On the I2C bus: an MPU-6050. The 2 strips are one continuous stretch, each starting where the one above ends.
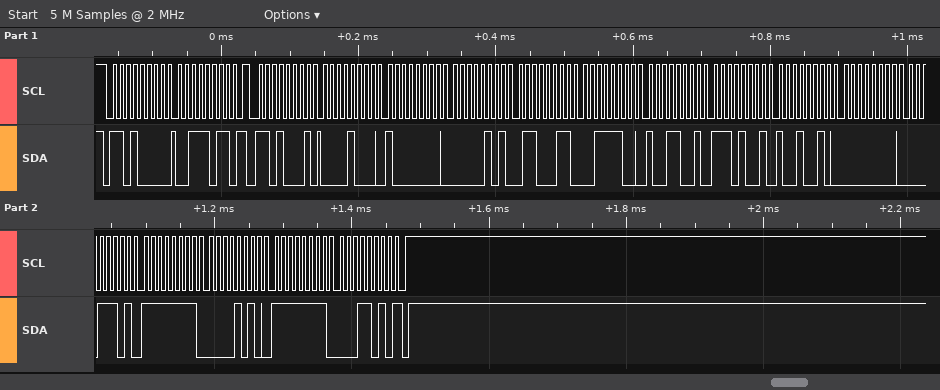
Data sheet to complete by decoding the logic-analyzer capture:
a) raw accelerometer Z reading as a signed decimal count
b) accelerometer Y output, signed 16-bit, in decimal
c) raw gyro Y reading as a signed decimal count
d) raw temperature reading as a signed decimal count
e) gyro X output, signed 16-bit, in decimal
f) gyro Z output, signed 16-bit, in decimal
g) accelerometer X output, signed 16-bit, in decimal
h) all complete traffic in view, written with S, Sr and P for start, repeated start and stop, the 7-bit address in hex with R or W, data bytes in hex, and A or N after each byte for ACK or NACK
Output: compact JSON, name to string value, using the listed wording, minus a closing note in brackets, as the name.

{"raw accelerometer Z reading as a signed decimal count": "15513", "accelerometer Y output, signed 16-bit, in decimal": "1379", "raw gyro Y reading as a signed decimal count": "-246", "raw temperature reading as a signed decimal count": "-5742", "gyro X output, signed 16-bit, in decimal": "29", "gyro Z output, signed 16-bit, in decimal": "-230", "accelerometer X output, signed 16-bit, in decimal": "2176", "all complete traffic in view, written with S, Sr and P for start, repeated start and stop, the 7-bit address in hex with R or W, data bytes in hex, and A or N after each byte for ACK or NACK": "S 68W A 3B A Sr 68R A 08 A 80 A 05 A 63 A 3C A 99 A E9 A 92 A 00 A 1D A FF A 0A A FF A 1A N P"}
